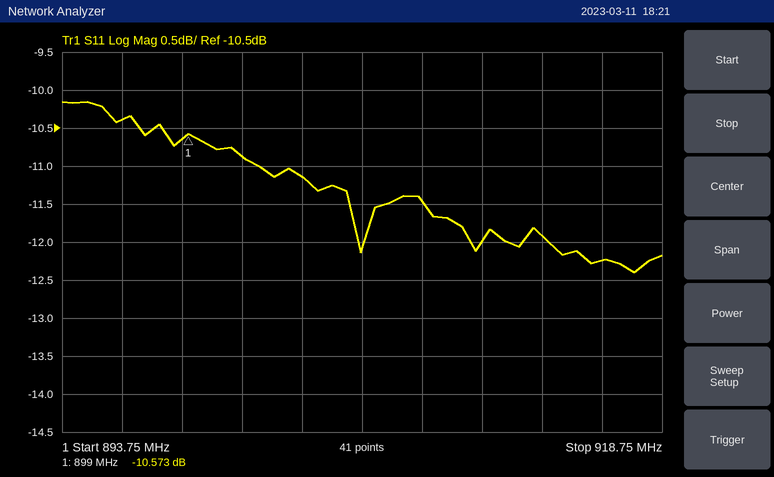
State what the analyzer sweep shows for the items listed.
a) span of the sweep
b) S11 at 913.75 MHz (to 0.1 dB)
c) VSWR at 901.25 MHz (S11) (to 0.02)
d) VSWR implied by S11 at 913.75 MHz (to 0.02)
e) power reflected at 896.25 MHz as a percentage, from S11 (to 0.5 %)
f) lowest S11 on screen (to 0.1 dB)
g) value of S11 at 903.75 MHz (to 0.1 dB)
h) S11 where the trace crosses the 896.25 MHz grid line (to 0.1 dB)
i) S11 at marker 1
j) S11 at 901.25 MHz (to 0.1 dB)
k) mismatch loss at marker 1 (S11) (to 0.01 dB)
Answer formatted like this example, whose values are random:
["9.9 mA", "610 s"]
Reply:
["25 MHz", "-11.9 dB", "1.80", "1.68", "9.0 %", "-12.4 dB", "-11.1 dB", "-10.4 dB", "-10.573 dB", "-10.9 dB", "0.40 dB"]
